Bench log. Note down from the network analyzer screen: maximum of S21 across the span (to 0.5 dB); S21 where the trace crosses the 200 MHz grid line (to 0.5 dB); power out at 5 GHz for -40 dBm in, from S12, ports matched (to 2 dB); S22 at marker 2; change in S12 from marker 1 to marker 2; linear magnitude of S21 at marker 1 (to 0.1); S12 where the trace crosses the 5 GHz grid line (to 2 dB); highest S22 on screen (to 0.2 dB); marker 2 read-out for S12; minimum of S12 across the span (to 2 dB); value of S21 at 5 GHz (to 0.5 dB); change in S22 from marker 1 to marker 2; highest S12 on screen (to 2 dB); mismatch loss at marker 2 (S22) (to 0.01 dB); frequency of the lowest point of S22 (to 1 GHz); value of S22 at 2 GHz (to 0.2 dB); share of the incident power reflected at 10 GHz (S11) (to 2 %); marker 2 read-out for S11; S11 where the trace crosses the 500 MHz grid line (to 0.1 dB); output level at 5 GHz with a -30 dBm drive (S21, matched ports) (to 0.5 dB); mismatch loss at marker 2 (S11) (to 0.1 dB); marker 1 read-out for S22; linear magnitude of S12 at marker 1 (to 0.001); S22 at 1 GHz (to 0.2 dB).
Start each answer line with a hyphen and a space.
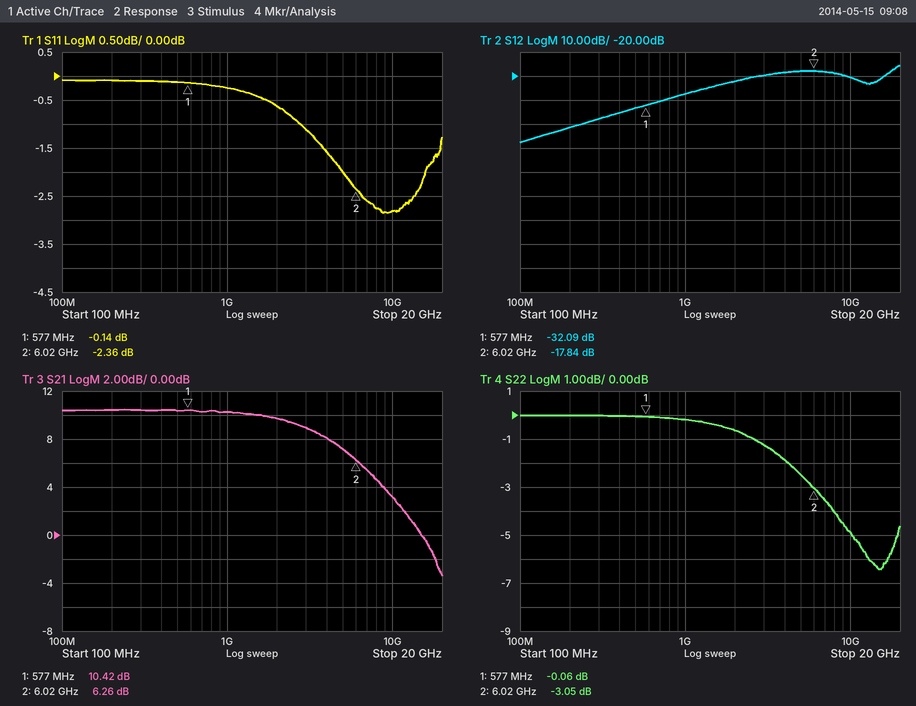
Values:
- 10.5 dB
- 10.5 dB
- -58 dBm
- -3.05 dB
- 14.25 dB
- 3.3
- -18 dB
- 0.0 dB
- -17.84 dB
- -48 dB
- 7.0 dB
- -2.99 dB
- -16 dB
- 2.97 dB
- 15 GHz
- -0.6 dB
- 52 %
- -2.36 dB
- -0.1 dB
- -23.0 dBm
- 3.8 dB
- -0.06 dB
- 0.025
- -0.2 dB
